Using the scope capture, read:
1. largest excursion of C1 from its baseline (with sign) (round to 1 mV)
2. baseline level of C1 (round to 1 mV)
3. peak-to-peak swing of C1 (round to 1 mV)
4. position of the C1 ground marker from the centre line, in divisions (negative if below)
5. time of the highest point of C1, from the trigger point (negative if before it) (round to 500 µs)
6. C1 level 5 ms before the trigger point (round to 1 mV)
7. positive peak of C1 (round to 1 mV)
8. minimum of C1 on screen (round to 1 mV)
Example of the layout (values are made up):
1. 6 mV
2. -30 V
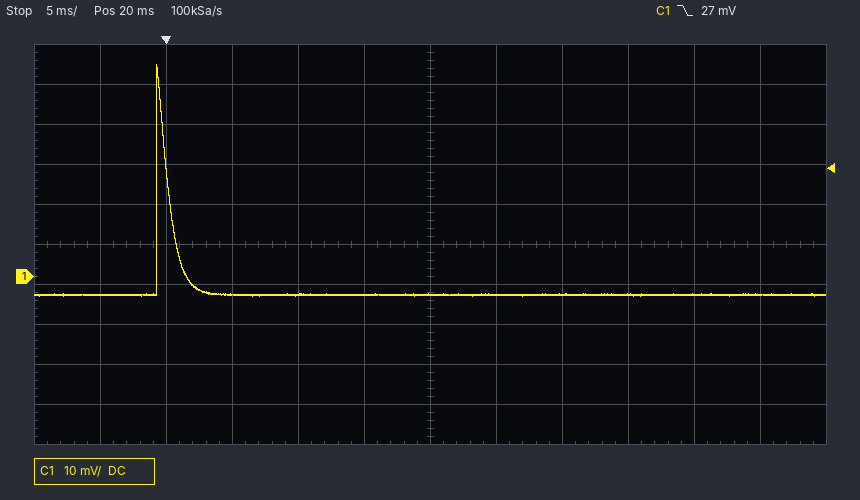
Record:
1. +58 mV
2. -5 mV
3. 58 mV
4. -0.8 div
5. -500 µs
6. -5 mV
7. 53 mV
8. -5 mV
